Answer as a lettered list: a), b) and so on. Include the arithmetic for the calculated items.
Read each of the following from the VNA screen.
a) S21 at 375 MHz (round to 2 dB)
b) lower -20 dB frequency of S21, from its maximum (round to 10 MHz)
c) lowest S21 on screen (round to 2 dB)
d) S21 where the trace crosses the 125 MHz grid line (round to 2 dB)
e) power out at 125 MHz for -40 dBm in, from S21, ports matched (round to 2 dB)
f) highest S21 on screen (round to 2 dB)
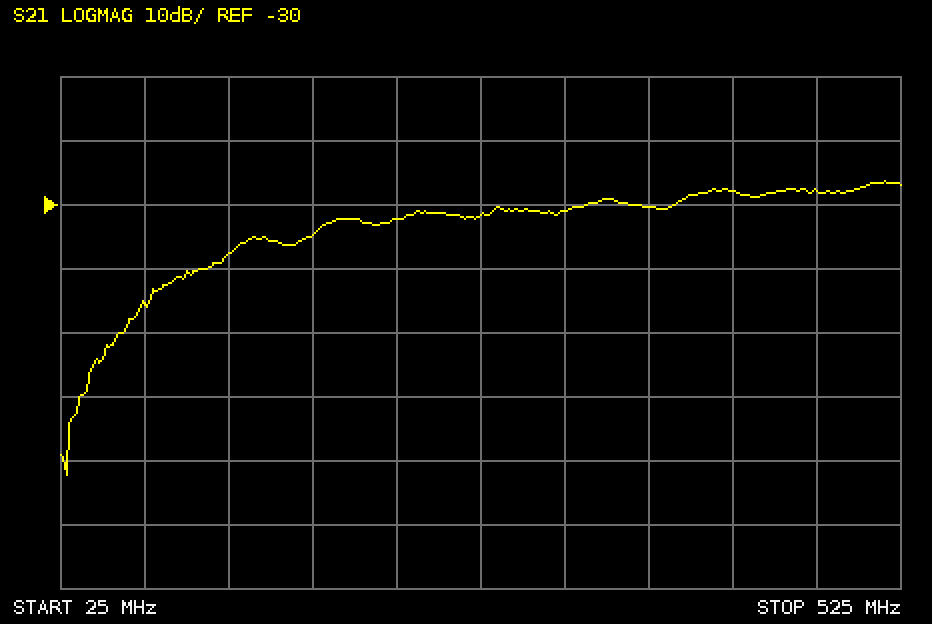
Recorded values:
a) -30 dB
b) 70 MHz
c) -72 dB
d) -38 dB
e) -40 dBm + (-38 dB) = -78 dBm
f) -26 dB
